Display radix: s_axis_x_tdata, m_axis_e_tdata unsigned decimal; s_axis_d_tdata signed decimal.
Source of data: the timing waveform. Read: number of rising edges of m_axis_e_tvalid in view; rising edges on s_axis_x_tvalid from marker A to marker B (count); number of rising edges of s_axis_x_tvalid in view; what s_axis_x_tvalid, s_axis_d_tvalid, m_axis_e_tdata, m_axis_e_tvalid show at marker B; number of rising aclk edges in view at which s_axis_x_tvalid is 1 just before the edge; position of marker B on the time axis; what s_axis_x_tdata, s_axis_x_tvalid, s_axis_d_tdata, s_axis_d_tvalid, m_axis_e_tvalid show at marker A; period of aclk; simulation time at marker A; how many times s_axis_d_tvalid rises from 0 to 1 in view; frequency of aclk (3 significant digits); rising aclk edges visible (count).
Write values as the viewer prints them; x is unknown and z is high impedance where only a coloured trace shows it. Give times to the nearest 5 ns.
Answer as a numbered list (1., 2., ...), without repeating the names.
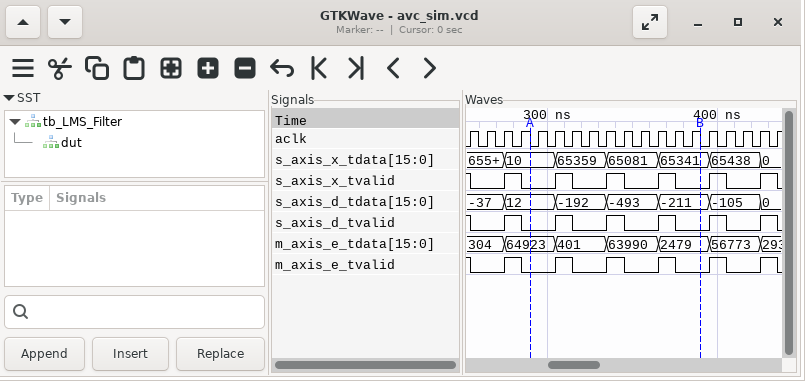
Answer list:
1. 6
2. 3
3. 6
4. s_axis_x_tvalid=0, s_axis_d_tvalid=0, m_axis_e_tdata=2479, m_axis_e_tvalid=0
5. 7
6. 390 ns
7. s_axis_x_tdata=10, s_axis_x_tvalid=0, s_axis_d_tdata=12, s_axis_d_tvalid=0, m_axis_e_tvalid=0
8. 10 ns
9. 290 ns
10. 6
11. 100 MHz
12. 19
